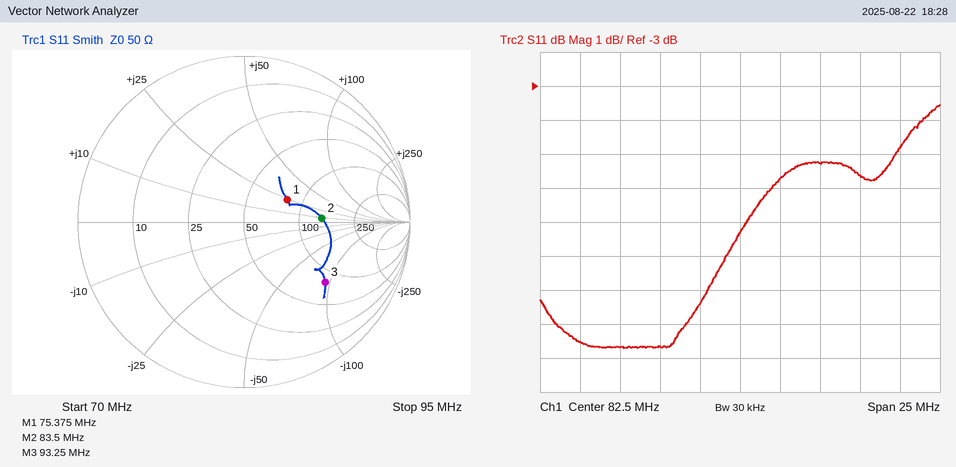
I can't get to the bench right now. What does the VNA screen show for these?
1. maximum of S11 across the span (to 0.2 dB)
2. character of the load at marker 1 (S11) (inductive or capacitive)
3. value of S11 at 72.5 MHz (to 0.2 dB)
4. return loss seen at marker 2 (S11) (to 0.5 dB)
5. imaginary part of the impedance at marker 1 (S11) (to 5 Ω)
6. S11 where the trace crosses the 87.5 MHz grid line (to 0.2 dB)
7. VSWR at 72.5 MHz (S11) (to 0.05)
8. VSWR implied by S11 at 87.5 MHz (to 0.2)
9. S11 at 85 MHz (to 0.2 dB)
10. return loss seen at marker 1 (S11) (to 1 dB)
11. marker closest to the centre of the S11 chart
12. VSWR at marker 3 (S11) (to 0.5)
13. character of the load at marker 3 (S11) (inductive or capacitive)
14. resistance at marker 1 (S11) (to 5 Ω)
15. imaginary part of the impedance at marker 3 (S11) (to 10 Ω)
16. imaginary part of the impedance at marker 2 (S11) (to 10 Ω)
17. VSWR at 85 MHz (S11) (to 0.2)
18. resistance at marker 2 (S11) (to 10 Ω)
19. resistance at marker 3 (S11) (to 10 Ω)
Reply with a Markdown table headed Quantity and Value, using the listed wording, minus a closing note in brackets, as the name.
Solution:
| Quantity | Value |
|---|---|
| maximum of S11 across the span | -3.6 dB |
| character of the load at marker 1 (S11) | inductive |
| value of S11 at 72.5 MHz | -10.6 dB |
| return loss seen at marker 2 (S11) | 6.5 dB |
| imaginary part of the impedance at marker 1 (S11) | +25 Ω |
| S11 where the trace crosses the 87.5 MHz grid line | -5.2 dB |
| VSWR at 72.5 MHz (S11) | 1.85 |
| VSWR implied by S11 at 87.5 MHz | 3.4 |
| S11 at 85 MHz | -5.8 dB |
| return loss seen at marker 1 (S11) | 11 dB |
| marker closest to the centre of the S11 chart | marker 1 |
| VSWR at marker 3 (S11) | 4.0 |
| character of the load at marker 3 (S11) | capacitive |
| resistance at marker 1 (S11) | 80 Ω |
| imaginary part of the impedance at marker 3 (S11) | -90 Ω |
| imaginary part of the impedance at marker 2 (S11) | +10 Ω |
| VSWR at 85 MHz (S11) | 3.2 |
| resistance at marker 2 (S11) | 140 Ω |
| resistance at marker 3 (S11) | 80 Ω |
